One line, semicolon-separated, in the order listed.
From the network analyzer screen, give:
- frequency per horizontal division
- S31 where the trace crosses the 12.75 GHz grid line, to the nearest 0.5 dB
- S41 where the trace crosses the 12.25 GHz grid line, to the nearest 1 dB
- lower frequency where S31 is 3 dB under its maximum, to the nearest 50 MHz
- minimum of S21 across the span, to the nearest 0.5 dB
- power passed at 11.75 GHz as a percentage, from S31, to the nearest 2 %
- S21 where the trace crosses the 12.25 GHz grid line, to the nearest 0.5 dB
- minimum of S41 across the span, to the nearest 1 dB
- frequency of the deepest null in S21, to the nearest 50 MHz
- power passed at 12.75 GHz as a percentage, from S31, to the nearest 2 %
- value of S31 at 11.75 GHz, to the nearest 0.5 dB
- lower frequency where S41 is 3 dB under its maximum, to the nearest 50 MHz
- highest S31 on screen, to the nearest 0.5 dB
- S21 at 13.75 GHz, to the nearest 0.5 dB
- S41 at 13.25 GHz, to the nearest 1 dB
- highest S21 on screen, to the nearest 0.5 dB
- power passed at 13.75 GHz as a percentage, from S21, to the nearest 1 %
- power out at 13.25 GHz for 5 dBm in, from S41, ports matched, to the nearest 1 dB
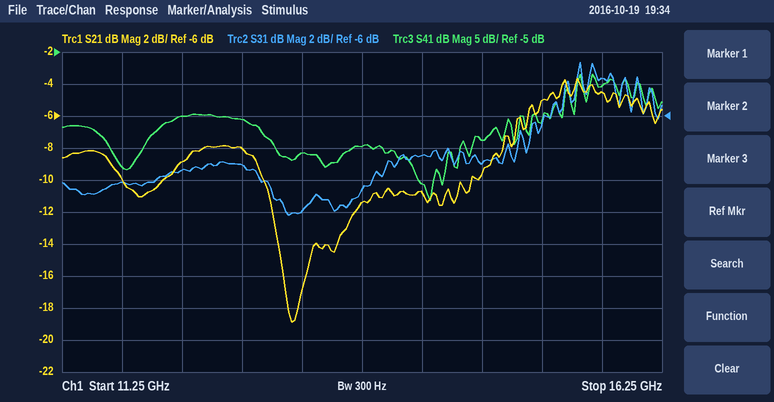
500 MHz; -9.0 dB; -15 dB; 15.40 GHz; -19.0 dB; 10 %; -9.0 dB; -28 dB; 13.15 GHz; 12 %; -10.0 dB; 15.55 GHz; -2.5 dB; -11.5 dB; -21 dB; -3.5 dB; 7 %; -16 dBm
